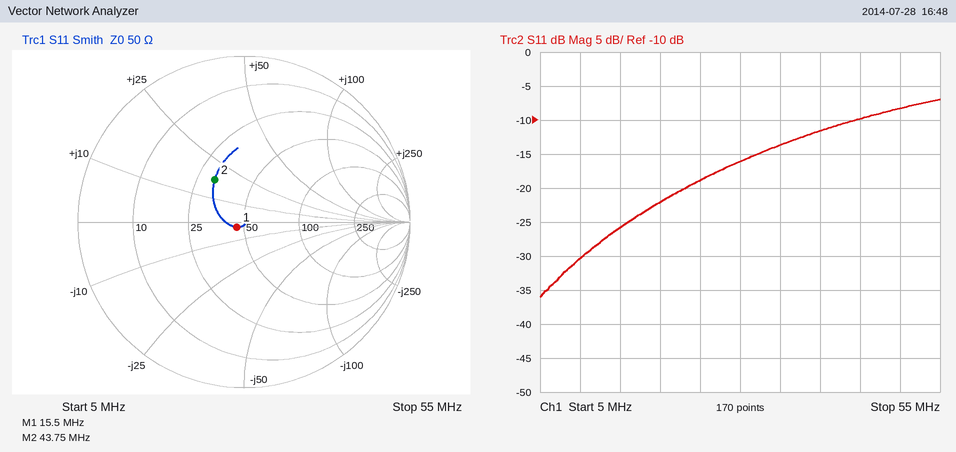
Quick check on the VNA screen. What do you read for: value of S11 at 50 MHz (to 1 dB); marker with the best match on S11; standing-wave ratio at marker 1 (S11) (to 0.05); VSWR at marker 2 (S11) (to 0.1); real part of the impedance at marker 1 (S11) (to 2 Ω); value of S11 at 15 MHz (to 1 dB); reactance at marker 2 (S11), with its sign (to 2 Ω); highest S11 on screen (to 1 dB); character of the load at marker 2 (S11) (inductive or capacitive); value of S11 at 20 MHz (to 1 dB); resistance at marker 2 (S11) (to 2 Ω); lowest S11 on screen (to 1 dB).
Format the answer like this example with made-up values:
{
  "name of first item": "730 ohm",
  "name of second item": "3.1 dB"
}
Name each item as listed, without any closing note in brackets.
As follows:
{
  "value of S11 at 50 MHz": "-8 dB",
  "marker with the best match on S11": "marker 1",
  "standing-wave ratio at marker 1 (S11)": "1.10",
  "VSWR at marker 2 (S11)": "1.9",
  "real part of the impedance at marker 1 (S11)": "46 Ω",
  "value of S11 at 15 MHz": "-26 dB",
  "reactance at marker 2 (S11), with its sign": "+18 Ω",
  "highest S11 on screen": "-7 dB",
  "character of the load at marker 2 (S11)": "inductive",
  "value of S11 at 20 MHz": "-22 dB",
  "resistance at marker 2 (S11)": "32 Ω",
  "lowest S11 on screen": "-36 dB"
}
